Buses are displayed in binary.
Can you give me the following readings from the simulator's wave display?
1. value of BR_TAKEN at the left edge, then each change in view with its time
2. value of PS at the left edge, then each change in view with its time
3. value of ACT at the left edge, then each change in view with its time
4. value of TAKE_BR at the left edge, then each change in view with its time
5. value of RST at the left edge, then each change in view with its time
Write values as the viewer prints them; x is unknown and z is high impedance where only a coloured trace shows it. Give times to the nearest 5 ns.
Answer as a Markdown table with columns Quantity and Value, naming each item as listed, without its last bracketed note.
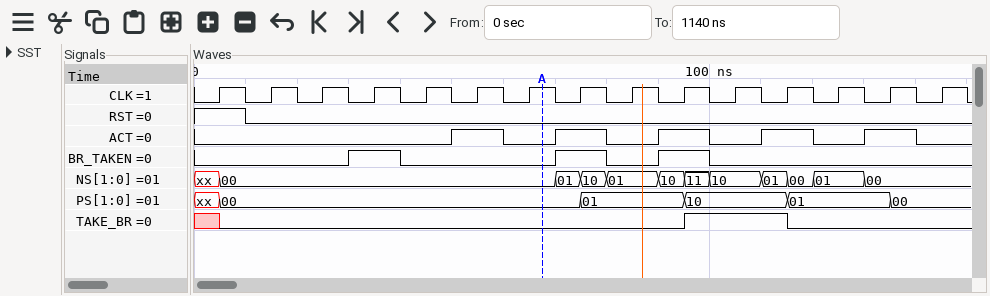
| Quantity | Value |
|---|---|
| value of BR_TAKEN at the left edge, then each change in view with its time | 0, 1 at 30 ns, 0 at 40 ns, 1 at 70 ns, 0 at 80 ns, 1 at 90 ns, 0 at 100 ns |
| value of PS at the left edge, then each change in view with its time | xx, 00 at 5 ns, 01 at 75 ns, 10 at 95 ns, 01 at 115 ns, 00 at 135 ns |
| value of ACT at the left edge, then each change in view with its time | 0, 1 at 50 ns, 0 at 60 ns, 1 at 70 ns, 0 at 80 ns, 1 at 90 ns, 0 at 100 ns, 1 at 110 ns, 0 at 120 ns, 1 at 130 ns, 0 at 140 ns |
| value of TAKE_BR at the left edge, then each change in view with its time | x, 0 at 5 ns, 1 at 95 ns, 0 at 115 ns |
| value of RST at the left edge, then each change in view with its time | 1, 0 at 10 ns |
